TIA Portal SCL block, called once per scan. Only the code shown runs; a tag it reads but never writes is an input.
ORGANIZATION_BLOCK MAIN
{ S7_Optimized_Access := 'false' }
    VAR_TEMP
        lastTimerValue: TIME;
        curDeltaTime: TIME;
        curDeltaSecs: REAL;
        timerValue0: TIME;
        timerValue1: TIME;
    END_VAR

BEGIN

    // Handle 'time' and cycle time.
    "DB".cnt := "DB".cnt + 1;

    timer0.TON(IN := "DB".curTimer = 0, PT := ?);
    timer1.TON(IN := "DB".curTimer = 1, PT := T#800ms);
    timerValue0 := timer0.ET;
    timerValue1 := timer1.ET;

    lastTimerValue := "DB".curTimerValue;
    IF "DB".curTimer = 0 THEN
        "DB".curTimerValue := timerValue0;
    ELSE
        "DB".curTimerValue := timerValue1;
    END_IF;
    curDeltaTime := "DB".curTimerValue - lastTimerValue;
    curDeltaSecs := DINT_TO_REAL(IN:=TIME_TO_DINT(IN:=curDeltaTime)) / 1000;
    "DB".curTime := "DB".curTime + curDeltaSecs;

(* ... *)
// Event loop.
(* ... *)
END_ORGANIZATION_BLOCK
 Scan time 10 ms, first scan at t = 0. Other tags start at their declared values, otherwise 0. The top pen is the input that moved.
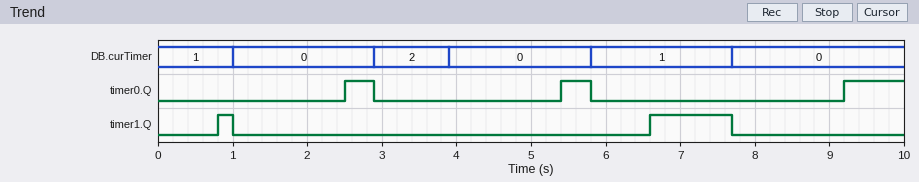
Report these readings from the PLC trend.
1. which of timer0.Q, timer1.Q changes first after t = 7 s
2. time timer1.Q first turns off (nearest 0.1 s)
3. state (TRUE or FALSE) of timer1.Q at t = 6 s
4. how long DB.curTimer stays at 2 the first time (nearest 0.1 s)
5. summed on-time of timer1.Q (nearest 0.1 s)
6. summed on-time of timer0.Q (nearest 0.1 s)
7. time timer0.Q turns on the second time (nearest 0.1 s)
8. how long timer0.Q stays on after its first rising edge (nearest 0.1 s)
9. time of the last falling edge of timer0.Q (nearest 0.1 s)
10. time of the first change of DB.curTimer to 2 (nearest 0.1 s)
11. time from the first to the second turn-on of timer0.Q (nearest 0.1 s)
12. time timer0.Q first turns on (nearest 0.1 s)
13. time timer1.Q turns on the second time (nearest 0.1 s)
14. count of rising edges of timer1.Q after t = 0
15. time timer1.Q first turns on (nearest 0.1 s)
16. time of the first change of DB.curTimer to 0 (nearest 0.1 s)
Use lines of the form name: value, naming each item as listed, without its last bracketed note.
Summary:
which of timer0.Q, timer1.Q changes first after t = 7 s: timer1.Q
time timer1.Q first turns off: 1.0 s
state (TRUE or FALSE) of timer1.Q at t = 6 s: FALSE
how long DB.curTimer stays at 2 the first time: 1.0 s
summed on-time of timer1.Q: 1.3 s
summed on-time of timer0.Q: 1.6 s
time timer0.Q turns on the second time: 5.4 s
how long timer0.Q stays on after its first rising edge: 0.4 s
time of the last falling edge of timer0.Q: 5.8 s
time of the first change of DB.curTimer to 2: 2.9 s
time from the first to the second turn-on of timer0.Q: 2.9 s
time timer0.Q first turns on: 2.5 s
time timer1.Q turns on the second time: 6.6 s
count of rising edges of timer1.Q after t = 0: 2
time timer1.Q first turns on: 0.8 s
time of the first change of DB.curTimer to 0: 1.0 s
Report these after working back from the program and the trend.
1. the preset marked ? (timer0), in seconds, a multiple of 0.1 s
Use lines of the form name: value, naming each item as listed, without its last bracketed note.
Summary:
the preset marked ? (timer0), in seconds, a multiple of 0.1 s: 1.5 s
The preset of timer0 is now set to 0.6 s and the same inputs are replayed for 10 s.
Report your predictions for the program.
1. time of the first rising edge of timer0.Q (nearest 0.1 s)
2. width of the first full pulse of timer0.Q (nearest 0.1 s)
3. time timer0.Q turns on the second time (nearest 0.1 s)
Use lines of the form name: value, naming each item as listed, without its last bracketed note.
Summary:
time of the first rising edge of timer0.Q: 1.6 s
width of the first full pulse of timer0.Q: 1.3 s
time timer0.Q turns on the second time: 4.5 s
